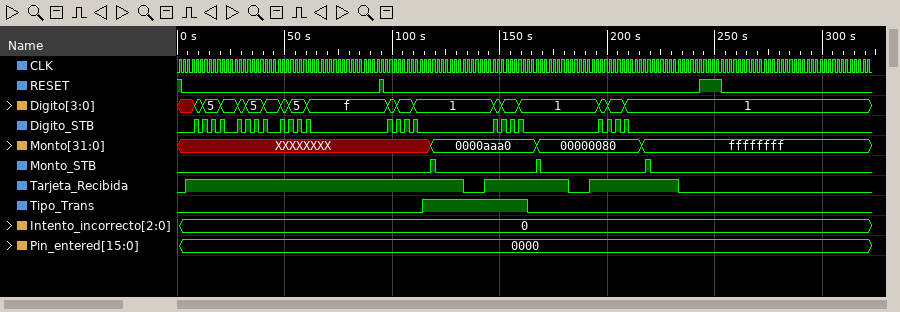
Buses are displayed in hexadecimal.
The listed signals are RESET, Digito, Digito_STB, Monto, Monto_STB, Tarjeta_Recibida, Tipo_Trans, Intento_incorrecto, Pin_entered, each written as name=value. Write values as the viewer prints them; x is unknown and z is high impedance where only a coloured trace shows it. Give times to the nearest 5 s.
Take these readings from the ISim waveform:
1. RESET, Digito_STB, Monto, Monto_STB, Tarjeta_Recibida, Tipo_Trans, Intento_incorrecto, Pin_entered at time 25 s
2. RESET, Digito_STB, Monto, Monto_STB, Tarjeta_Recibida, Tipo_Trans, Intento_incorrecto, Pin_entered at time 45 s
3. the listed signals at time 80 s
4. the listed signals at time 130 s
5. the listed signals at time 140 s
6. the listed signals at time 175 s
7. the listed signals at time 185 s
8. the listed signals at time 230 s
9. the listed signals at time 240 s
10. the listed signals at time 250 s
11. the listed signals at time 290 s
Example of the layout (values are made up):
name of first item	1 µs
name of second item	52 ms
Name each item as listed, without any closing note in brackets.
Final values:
RESET, Digito_STB, Monto, Monto_STB, Tarjeta_Recibida, Tipo_Trans, Intento_incorrecto, Pin_entered at time 25 s	RESET=0, Digito_STB=0, Monto=XXXXXXXX, Monto_STB=0, Tarjeta_Recibida=1, Tipo_Trans=0, Intento_incorrecto=0, Pin_entered=0000
RESET, Digito_STB, Monto, Monto_STB, Tarjeta_Recibida, Tipo_Trans, Intento_incorrecto, Pin_entered at time 45 s	RESET=0, Digito_STB=0, Monto=XXXXXXXX, Monto_STB=0, Tarjeta_Recibida=1, Tipo_Trans=0, Intento_incorrecto=0, Pin_entered=0000
the listed signals at time 80 s	RESET=0, Digito=f, Digito_STB=0, Monto=XXXXXXXX, Monto_STB=0, Tarjeta_Recibida=1, Tipo_Trans=0, Intento_incorrecto=0, Pin_entered=0000
the listed signals at time 130 s	RESET=0, Digito=1, Digito_STB=0, Monto=0000aaa0, Monto_STB=0, Tarjeta_Recibida=1, Tipo_Trans=1, Intento_incorrecto=0, Pin_entered=0000
the listed signals at time 140 s	RESET=0, Digito=1, Digito_STB=0, Monto=0000aaa0, Monto_STB=0, Tarjeta_Recibida=0, Tipo_Trans=1, Intento_incorrecto=0, Pin_entered=0000
the listed signals at time 175 s	RESET=0, Digito=1, Digito_STB=0, Monto=00000080, Monto_STB=0, Tarjeta_Recibida=1, Tipo_Trans=0, Intento_incorrecto=0, Pin_entered=0000
the listed signals at time 185 s	RESET=0, Digito=1, Digito_STB=0, Monto=00000080, Monto_STB=0, Tarjeta_Recibida=0, Tipo_Trans=0, Intento_incorrecto=0, Pin_entered=0000
the listed signals at time 230 s	RESET=0, Digito=1, Digito_STB=0, Monto=ffffffff, Monto_STB=0, Tarjeta_Recibida=1, Tipo_Trans=0, Intento_incorrecto=0, Pin_entered=0000
the listed signals at time 240 s	RESET=0, Digito=1, Digito_STB=0, Monto=ffffffff, Monto_STB=0, Tarjeta_Recibida=0, Tipo_Trans=0, Intento_incorrecto=0, Pin_entered=0000
the listed signals at time 250 s	RESET=1, Digito=1, Digito_STB=0, Monto=ffffffff, Monto_STB=0, Tarjeta_Recibida=0, Tipo_Trans=0, Intento_incorrecto=0, Pin_entered=0000
the listed signals at time 290 s	RESET=0, Digito=1, Digito_STB=0, Monto=ffffffff, Monto_STB=0, Tarjeta_Recibida=0, Tipo_Trans=0, Intento_incorrecto=0, Pin_entered=0000
